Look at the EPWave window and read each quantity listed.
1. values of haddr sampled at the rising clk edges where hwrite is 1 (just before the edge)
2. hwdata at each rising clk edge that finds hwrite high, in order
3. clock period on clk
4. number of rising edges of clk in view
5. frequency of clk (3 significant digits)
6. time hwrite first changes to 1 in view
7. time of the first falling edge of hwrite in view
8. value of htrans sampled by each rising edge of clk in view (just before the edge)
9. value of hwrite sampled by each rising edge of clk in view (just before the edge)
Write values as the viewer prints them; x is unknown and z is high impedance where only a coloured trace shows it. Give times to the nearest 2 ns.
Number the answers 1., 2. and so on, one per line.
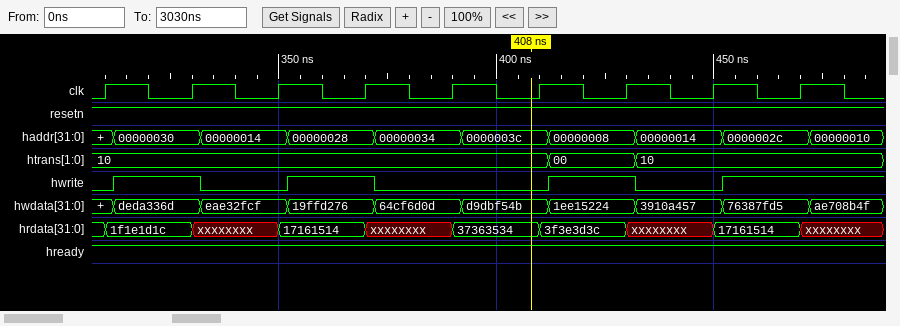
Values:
1. 00000030, 00000028, 00000008, 0000002c
2. deda336d, 19ffd276, 1ee15224, 76387fd5
3. 20 ns
4. 9
5. 50.0 MHz
6. 312 ns
7. 332 ns
8. 10, 10, 10, 10, 10, 10, 00, 10, 10
9. 0 1 0 1 0 0 1 0 1
